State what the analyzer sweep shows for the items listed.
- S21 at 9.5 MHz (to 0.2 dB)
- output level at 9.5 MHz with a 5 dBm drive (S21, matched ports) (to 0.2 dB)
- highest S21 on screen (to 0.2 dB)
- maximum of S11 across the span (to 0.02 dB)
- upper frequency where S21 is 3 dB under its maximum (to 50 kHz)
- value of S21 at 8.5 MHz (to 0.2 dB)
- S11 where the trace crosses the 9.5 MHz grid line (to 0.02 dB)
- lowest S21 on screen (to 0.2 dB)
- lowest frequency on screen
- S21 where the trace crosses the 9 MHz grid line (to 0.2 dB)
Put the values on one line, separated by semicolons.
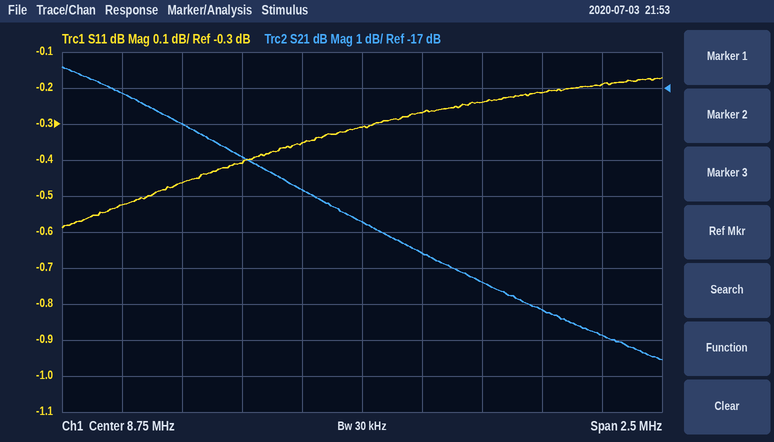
-23.2 dB; -18.2 dBm; -16.4 dB; -0.18 dB; 8.40 MHz; -19.8 dB; -0.22 dB; -24.6 dB; 7.5 MHz; -21.6 dB
